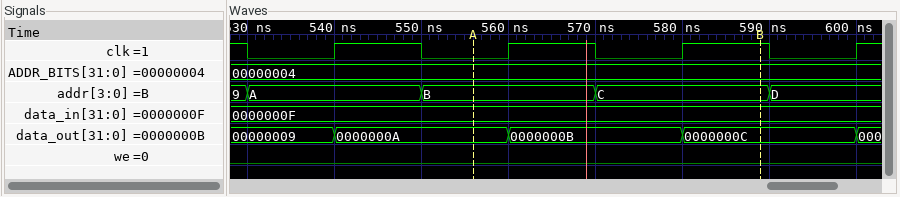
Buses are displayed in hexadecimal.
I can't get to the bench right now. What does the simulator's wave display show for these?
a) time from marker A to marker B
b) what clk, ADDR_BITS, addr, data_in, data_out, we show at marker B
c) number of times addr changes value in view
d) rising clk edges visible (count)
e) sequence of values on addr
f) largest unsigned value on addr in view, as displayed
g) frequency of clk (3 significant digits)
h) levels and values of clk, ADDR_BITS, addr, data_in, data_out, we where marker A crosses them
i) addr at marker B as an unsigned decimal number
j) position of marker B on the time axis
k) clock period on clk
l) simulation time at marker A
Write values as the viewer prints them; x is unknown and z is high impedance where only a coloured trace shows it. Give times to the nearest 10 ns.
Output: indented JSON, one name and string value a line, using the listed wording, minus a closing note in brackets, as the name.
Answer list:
{
  "time from marker A to marker B": "30 ns",
  "what clk, ADDR_BITS, addr, data_in, data_out, we show at marker B": "clk=1, ADDR_BITS=00000004, addr=C, data_in=0000000F, data_out=0000000C, we=0",
  "number of times addr changes value in view": "4",
  "rising clk edges visible": "4",
  "sequence of values on addr": "9, A, B, C, D",
  "largest unsigned value on addr in view, as displayed": "D",
  "frequency of clk": "50.0 MHz",
  "levels and values of clk, ADDR_BITS, addr, data_in, data_out, we where marker A crosses them": "clk=0, ADDR_BITS=00000004, addr=B, data_in=0000000F, data_out=0000000A, we=0",
  "addr at marker B as an unsigned decimal number": "12",
  "position of marker B on the time axis": "590 ns",
  "clock period on clk": "20 ns",
  "simulation time at marker A": "560 ns"
}
